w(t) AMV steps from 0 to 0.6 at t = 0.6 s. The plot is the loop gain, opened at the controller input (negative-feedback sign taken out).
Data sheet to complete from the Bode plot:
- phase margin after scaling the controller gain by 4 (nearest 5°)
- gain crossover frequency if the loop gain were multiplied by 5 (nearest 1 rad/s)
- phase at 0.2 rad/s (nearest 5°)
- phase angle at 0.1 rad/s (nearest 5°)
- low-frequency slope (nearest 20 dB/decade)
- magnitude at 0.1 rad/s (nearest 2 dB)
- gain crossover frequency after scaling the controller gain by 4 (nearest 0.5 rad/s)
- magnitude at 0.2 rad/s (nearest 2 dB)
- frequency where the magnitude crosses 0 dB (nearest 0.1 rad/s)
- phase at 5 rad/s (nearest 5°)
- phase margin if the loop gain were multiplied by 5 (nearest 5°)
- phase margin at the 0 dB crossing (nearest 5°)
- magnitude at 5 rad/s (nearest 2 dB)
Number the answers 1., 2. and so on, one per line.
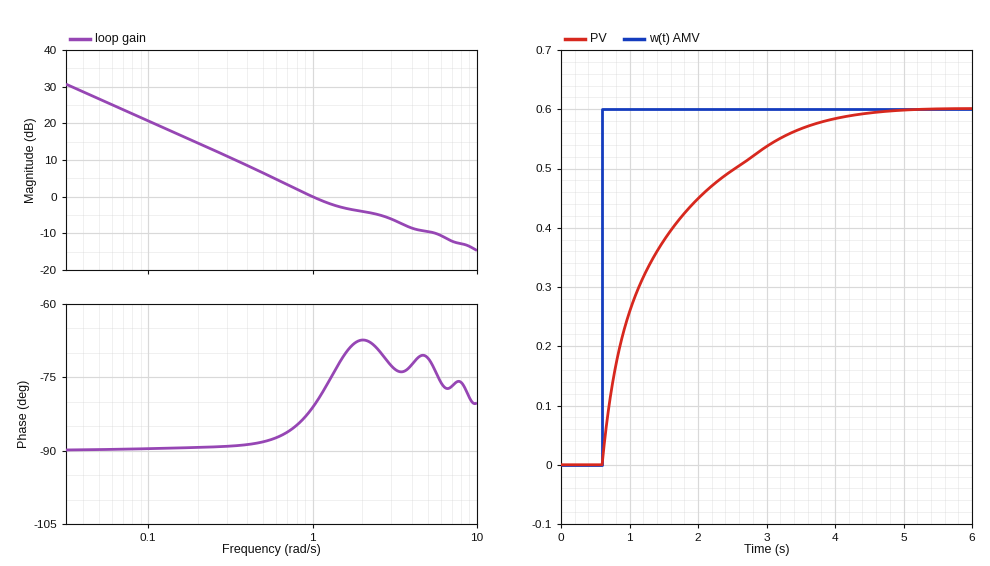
1. 105°
2. 9 rad/s
3. -90°
4. -90°
5. -20 dB/decade
6. 20 dB
7. 7.0 rad/s
8. 14 dB
9. 1.0 rad/s
10. -70°
11. 100°
12. 100°
13. -10 dB
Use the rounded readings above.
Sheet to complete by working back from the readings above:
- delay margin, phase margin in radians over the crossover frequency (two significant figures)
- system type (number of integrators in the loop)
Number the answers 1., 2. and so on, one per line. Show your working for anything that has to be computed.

1. 100 × π / 180 / 1 = 1.7 s
2. 1
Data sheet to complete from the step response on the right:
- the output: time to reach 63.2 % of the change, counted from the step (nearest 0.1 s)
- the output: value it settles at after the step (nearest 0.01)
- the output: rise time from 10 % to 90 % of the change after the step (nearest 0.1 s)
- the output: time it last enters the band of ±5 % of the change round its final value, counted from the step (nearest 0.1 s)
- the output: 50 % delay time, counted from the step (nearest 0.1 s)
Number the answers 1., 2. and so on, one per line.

1. 0.9 s
2. 0.60
3. 2.4 s
4. 3.0 s
5. 0.5 s
